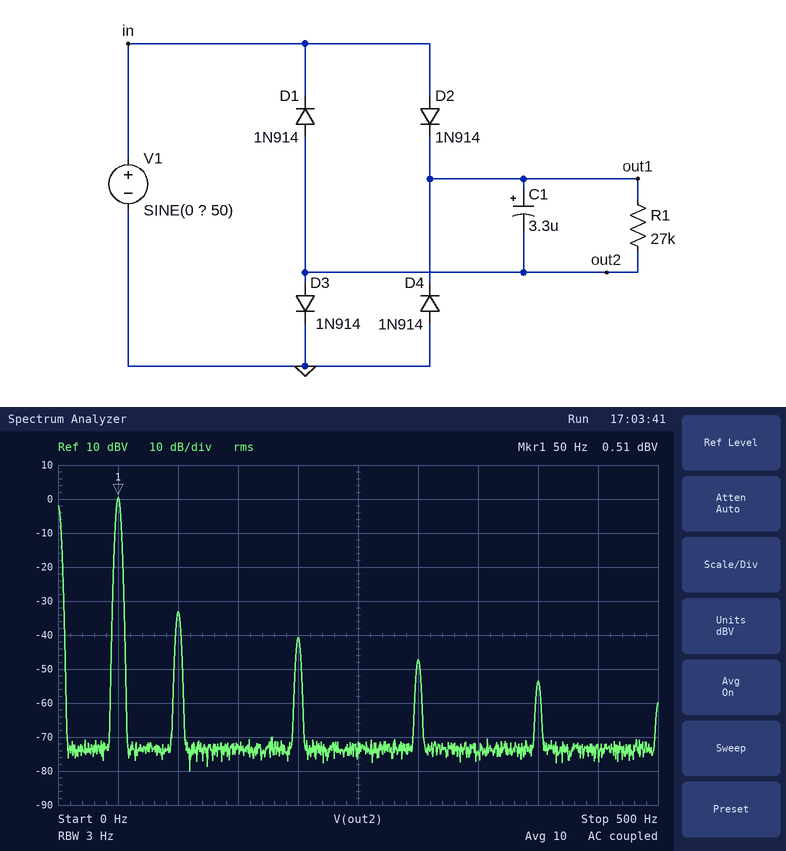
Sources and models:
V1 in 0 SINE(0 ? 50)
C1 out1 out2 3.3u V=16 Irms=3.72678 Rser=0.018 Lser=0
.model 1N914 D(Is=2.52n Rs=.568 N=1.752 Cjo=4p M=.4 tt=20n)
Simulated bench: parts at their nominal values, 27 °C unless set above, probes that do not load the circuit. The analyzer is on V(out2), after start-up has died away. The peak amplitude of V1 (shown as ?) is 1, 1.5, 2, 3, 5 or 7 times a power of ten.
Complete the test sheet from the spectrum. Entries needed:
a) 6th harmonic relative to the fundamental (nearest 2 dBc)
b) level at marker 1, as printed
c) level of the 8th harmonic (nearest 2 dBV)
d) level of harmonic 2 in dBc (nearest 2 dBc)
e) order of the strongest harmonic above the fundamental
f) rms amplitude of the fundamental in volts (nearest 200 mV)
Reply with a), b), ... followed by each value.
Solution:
a) -48 dBc
b) 0.51 dBV
c) -54 dBV
d) -34 dBc
e) 2
f) 1.0 V
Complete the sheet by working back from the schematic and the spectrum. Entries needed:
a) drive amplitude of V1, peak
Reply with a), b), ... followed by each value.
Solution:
a) 3 V
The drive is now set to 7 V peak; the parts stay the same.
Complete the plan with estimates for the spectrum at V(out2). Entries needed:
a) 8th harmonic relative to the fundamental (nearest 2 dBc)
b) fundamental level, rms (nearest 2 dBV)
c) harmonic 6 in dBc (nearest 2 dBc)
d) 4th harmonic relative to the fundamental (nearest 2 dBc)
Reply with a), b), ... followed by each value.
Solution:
a) -48 dBc
b) 8 dBV
c) -44 dBc
d) -38 dBc
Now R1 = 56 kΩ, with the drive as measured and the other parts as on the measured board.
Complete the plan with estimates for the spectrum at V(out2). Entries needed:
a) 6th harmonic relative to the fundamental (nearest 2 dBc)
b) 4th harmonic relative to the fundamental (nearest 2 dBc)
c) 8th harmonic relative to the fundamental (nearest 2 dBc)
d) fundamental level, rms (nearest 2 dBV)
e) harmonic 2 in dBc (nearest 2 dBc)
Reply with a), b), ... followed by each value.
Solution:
a) -54 dBc
b) -48 dBc
c) -60 dBc
d) 0 dBV
e) -40 dBc
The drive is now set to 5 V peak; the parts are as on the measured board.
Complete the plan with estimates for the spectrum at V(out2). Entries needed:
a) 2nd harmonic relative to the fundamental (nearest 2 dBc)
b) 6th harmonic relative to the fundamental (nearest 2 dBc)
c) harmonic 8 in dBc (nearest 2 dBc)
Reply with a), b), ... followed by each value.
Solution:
a) -32 dBc
b) -44 dBc
c) -50 dBc
